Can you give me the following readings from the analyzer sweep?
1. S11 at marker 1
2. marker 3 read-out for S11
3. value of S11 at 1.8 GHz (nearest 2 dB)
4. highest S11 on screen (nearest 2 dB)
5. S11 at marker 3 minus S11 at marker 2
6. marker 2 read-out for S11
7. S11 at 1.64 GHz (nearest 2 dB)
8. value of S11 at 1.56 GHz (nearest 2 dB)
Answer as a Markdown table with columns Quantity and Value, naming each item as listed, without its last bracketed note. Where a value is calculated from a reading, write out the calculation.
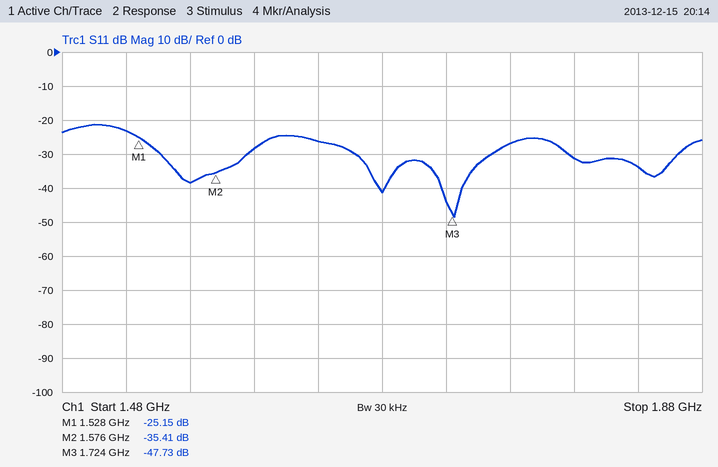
| Quantity | Value |
|---|---|
| S11 at marker 1 | -25.15 dB |
| marker 3 read-out for S11 | -47.73 dB |
| value of S11 at 1.8 GHz | -32 dB |
| highest S11 on screen | -22 dB |
| S11 at marker 3 minus S11 at marker 2 | -47.73 − (-35.41) = -12.32 dB |
| marker 2 read-out for S11 | -35.41 dB |
| S11 at 1.64 GHz | -26 dB |
| value of S11 at 1.56 GHz | -38 dB |
